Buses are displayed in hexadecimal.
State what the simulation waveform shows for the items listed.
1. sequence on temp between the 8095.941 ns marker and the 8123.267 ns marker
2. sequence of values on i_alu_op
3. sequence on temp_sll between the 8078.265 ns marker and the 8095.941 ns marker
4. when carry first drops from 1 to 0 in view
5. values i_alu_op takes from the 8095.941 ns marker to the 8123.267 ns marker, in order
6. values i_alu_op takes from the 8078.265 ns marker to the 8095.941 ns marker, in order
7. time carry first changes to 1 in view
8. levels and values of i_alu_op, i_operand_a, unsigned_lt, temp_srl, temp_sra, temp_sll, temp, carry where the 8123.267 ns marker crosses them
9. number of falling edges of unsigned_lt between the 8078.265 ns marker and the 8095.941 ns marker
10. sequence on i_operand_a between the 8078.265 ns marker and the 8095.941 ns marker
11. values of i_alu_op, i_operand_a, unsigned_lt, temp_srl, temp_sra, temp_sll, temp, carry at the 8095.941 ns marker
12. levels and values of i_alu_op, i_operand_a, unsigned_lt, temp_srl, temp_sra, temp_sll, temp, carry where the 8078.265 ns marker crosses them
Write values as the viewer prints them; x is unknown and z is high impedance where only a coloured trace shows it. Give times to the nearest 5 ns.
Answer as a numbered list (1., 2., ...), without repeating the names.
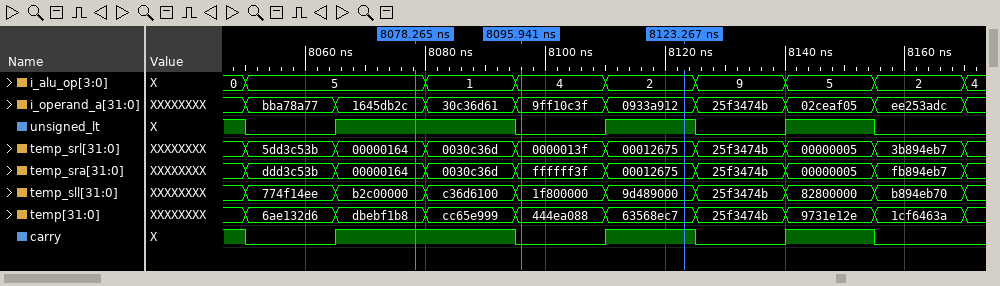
1. 444ea088, 63568ec7
2. 0, 5, 1, 4, 2, 9, 5, 2, 4
3. b2c00000, c36d6100, 1f800000
4. 8050 ns
5. 4, 2
6. 5, 1, 4
7. 8065 ns
8. i_alu_op=2, i_operand_a=0933a912, unsigned_lt=1, temp_srl=00012675, temp_sra=00012675, temp_sll=9d489000, temp=63568ec7, carry=1
9. 1
10. 1645db2c, 30c36d61, 9ff10c3f
11. i_alu_op=4, i_operand_a=9ff10c3f, unsigned_lt=0, temp_srl=0000013f, temp_sra=ffffff3f, temp_sll=1f800000, temp=444ea088, carry=0
12. i_alu_op=5, i_operand_a=1645db2c, unsigned_lt=1, temp_srl=00000164, temp_sra=00000164, temp_sll=b2c00000, temp=dbebf1b8, carry=1
